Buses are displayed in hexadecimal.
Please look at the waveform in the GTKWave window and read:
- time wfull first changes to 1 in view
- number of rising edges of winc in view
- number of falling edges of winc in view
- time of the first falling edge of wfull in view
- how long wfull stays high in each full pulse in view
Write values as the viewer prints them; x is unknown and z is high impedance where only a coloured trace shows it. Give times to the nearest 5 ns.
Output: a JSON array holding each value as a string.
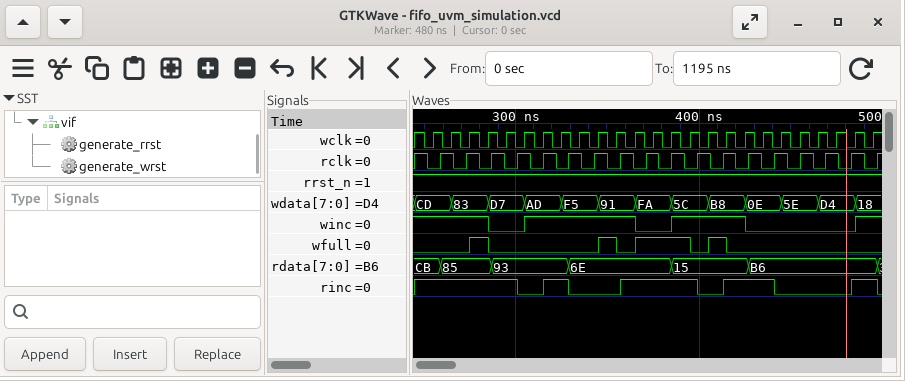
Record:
["275 ns", "3", "3", "285 ns", "10 ns, 10 ns, 30 ns, 10 ns"]
